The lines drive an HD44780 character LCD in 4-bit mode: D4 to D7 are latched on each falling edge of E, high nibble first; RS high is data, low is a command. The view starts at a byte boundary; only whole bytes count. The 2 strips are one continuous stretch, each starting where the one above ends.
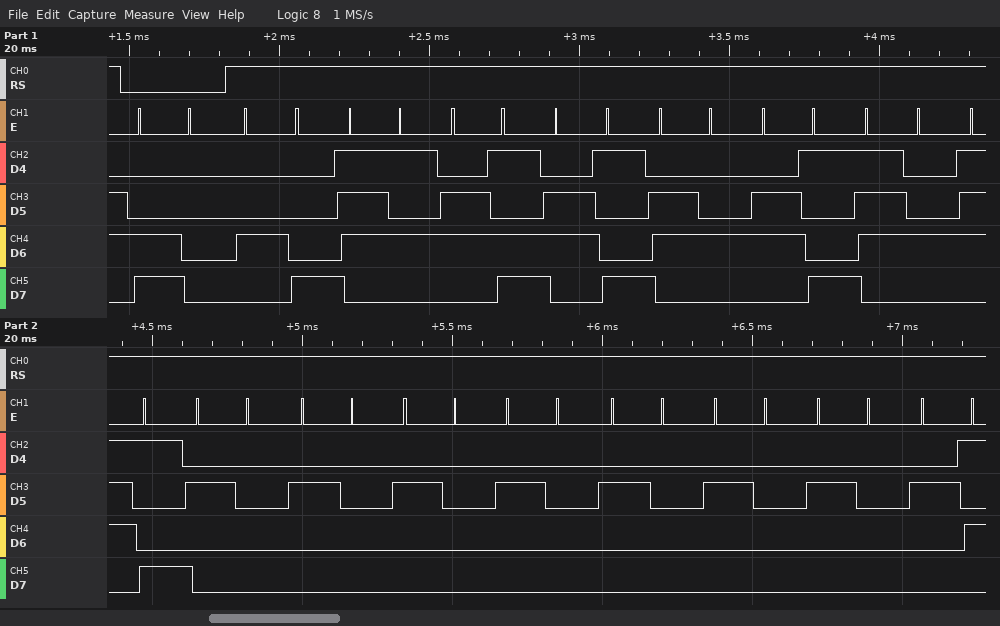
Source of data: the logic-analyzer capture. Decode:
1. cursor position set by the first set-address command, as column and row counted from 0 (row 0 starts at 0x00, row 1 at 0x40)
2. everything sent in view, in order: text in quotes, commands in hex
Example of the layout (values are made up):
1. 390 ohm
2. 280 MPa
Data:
1. column 0, row 1
2. 0xC0 "Humidity       %"
